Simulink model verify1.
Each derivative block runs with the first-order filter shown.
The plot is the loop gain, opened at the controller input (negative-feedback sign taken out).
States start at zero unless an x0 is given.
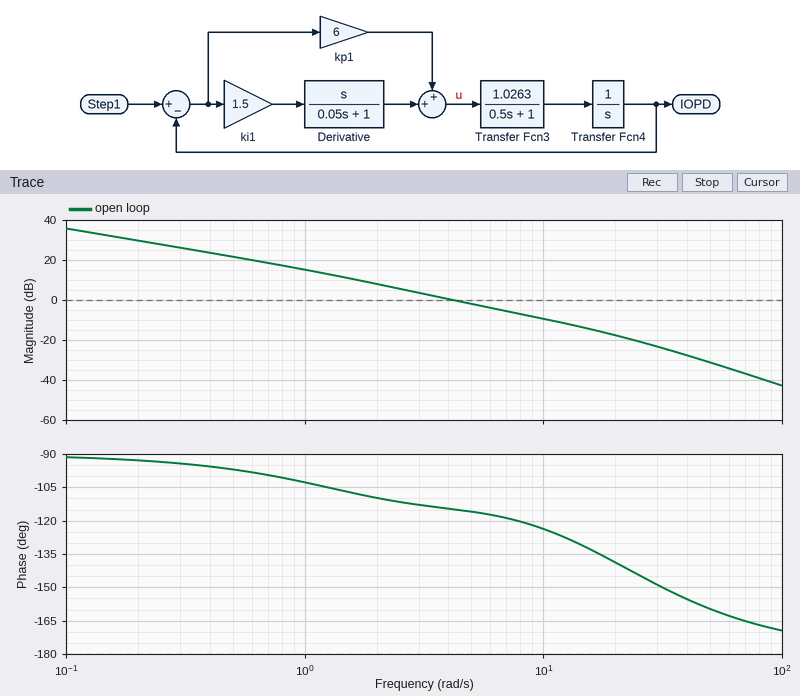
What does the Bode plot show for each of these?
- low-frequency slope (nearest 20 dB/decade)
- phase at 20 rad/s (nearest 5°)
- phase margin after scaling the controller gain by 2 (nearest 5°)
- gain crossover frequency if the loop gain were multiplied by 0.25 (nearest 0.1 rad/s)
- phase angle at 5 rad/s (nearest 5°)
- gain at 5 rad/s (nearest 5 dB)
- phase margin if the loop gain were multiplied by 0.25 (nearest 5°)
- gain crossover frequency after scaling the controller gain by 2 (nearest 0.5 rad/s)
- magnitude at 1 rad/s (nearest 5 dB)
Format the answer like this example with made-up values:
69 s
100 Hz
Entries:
-20 dB/decade
-140°
60°
1.4 rad/s
-115°
0 dB
75°
7.5 rad/s
15 dB
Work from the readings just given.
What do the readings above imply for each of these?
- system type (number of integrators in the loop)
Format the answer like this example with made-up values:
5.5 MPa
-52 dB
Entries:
1
